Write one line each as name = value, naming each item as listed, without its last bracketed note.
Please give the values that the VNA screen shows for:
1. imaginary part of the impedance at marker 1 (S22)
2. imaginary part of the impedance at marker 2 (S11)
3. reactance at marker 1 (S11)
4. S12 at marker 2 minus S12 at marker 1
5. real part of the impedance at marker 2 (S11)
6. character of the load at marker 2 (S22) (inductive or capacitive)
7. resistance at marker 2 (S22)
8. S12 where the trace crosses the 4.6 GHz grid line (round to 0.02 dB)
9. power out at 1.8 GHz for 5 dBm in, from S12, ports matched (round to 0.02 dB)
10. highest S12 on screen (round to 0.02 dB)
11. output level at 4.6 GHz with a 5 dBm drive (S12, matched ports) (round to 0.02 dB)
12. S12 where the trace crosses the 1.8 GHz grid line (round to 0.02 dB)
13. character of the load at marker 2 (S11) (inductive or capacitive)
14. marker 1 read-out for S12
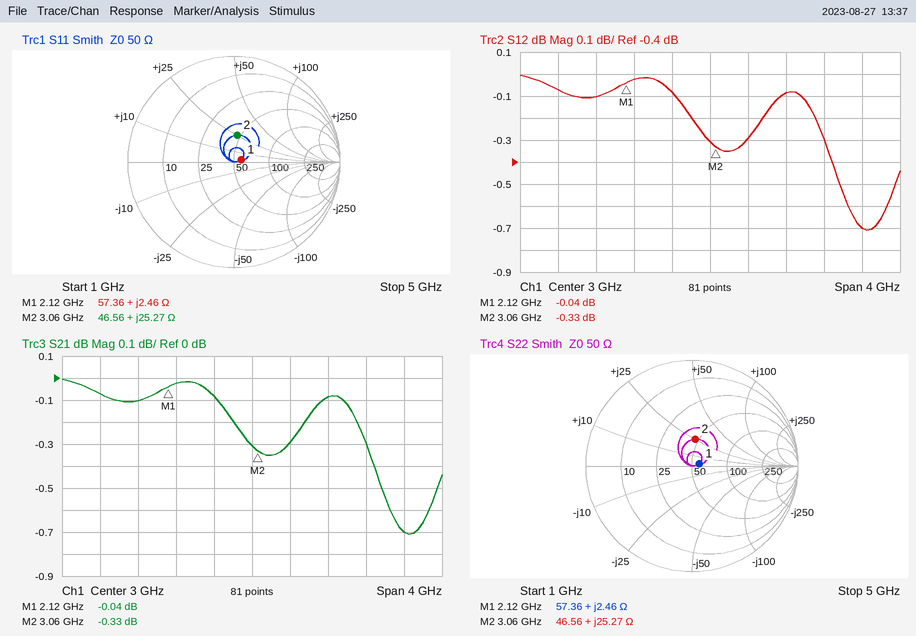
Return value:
imaginary part of the impedance at marker 1 = +2.46 Ω
imaginary part of the impedance at marker 2 = +25.27 Ω
reactance at marker 1 = +2.46 Ω
S12 at marker 2 minus S12 at marker 1 = -0.29 dB
real part of the impedance at marker 2 = 46.56 Ω
character of the load at marker 2 (S22) = inductive
resistance at marker 2 = 46.56 Ω
S12 where the trace crosses the 4.6 GHz grid line = -0.70 dB
power out at 1.8 GHz for 5 dBm in, from S12, ports matched = 4.90 dBm
highest S12 on screen = 0.00 dB
output level at 4.6 GHz with a 5 dBm drive (S12, matched ports) = 4.30 dBm
S12 where the trace crosses the 1.8 GHz grid line = -0.10 dB
character of the load at marker 2 (S11) = inductive
marker 1 read-out for S12 = -0.04 dB
